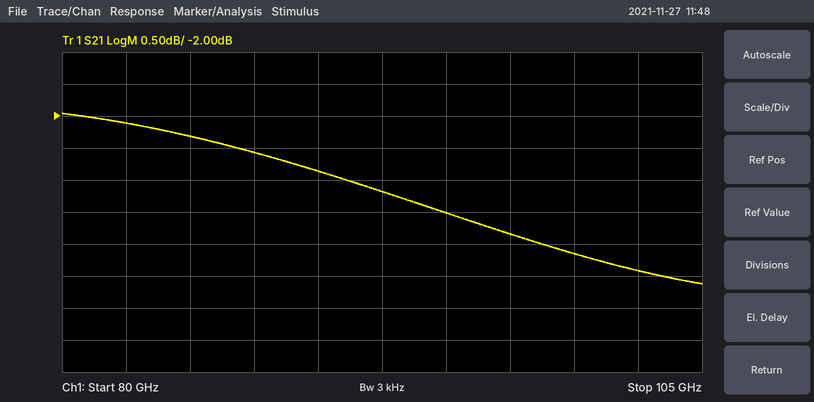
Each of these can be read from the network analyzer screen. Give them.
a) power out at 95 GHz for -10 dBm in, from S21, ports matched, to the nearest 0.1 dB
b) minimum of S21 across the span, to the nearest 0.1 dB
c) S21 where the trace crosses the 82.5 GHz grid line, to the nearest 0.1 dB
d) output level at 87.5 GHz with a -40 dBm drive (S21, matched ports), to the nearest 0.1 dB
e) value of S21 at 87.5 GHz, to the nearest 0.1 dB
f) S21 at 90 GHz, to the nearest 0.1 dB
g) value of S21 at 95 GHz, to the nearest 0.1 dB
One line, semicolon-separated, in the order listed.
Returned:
-13.5 dBm; -4.6 dB; -2.1 dB; -42.6 dBm; -2.6 dB; -2.9 dB; -3.5 dB
